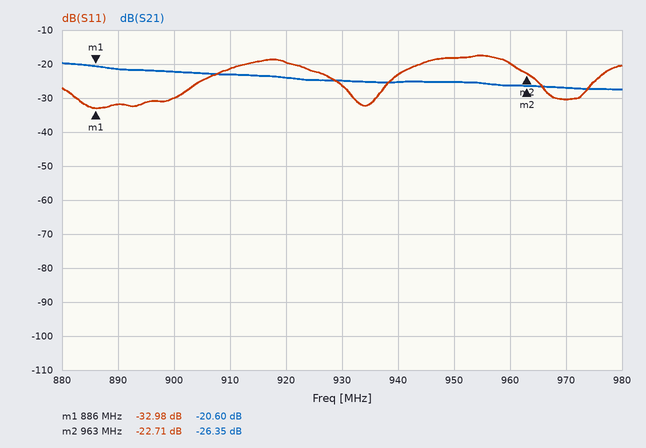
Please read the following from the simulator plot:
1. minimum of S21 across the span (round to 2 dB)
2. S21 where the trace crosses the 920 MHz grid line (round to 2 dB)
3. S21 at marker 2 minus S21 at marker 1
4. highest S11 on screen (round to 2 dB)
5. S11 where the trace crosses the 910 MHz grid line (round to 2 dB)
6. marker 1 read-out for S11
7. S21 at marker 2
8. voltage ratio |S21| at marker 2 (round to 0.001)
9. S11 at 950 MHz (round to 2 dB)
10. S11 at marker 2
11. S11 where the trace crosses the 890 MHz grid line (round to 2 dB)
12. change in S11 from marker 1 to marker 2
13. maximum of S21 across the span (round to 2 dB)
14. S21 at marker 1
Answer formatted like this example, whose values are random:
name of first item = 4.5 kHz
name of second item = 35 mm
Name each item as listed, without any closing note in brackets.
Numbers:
minimum of S21 across the span = -28 dB
S21 where the trace crosses the 920 MHz grid line = -24 dB
S21 at marker 2 minus S21 at marker 1 = -5.75 dB
highest S11 on screen = -18 dB
S11 where the trace crosses the 910 MHz grid line = -22 dB
marker 1 read-out for S11 = -32.98 dB
S21 at marker 2 = -26.35 dB
voltage ratio |S21| at marker 2 = 0.048
S11 at 950 MHz = -18 dB
S11 at marker 2 = -22.71 dB
S11 where the trace crosses the 890 MHz grid line = -32 dB
change in S11 from marker 1 to marker 2 = 10.27 dB
maximum of S21 across the span = -20 dB
S21 at marker 1 = -20.60 dB
